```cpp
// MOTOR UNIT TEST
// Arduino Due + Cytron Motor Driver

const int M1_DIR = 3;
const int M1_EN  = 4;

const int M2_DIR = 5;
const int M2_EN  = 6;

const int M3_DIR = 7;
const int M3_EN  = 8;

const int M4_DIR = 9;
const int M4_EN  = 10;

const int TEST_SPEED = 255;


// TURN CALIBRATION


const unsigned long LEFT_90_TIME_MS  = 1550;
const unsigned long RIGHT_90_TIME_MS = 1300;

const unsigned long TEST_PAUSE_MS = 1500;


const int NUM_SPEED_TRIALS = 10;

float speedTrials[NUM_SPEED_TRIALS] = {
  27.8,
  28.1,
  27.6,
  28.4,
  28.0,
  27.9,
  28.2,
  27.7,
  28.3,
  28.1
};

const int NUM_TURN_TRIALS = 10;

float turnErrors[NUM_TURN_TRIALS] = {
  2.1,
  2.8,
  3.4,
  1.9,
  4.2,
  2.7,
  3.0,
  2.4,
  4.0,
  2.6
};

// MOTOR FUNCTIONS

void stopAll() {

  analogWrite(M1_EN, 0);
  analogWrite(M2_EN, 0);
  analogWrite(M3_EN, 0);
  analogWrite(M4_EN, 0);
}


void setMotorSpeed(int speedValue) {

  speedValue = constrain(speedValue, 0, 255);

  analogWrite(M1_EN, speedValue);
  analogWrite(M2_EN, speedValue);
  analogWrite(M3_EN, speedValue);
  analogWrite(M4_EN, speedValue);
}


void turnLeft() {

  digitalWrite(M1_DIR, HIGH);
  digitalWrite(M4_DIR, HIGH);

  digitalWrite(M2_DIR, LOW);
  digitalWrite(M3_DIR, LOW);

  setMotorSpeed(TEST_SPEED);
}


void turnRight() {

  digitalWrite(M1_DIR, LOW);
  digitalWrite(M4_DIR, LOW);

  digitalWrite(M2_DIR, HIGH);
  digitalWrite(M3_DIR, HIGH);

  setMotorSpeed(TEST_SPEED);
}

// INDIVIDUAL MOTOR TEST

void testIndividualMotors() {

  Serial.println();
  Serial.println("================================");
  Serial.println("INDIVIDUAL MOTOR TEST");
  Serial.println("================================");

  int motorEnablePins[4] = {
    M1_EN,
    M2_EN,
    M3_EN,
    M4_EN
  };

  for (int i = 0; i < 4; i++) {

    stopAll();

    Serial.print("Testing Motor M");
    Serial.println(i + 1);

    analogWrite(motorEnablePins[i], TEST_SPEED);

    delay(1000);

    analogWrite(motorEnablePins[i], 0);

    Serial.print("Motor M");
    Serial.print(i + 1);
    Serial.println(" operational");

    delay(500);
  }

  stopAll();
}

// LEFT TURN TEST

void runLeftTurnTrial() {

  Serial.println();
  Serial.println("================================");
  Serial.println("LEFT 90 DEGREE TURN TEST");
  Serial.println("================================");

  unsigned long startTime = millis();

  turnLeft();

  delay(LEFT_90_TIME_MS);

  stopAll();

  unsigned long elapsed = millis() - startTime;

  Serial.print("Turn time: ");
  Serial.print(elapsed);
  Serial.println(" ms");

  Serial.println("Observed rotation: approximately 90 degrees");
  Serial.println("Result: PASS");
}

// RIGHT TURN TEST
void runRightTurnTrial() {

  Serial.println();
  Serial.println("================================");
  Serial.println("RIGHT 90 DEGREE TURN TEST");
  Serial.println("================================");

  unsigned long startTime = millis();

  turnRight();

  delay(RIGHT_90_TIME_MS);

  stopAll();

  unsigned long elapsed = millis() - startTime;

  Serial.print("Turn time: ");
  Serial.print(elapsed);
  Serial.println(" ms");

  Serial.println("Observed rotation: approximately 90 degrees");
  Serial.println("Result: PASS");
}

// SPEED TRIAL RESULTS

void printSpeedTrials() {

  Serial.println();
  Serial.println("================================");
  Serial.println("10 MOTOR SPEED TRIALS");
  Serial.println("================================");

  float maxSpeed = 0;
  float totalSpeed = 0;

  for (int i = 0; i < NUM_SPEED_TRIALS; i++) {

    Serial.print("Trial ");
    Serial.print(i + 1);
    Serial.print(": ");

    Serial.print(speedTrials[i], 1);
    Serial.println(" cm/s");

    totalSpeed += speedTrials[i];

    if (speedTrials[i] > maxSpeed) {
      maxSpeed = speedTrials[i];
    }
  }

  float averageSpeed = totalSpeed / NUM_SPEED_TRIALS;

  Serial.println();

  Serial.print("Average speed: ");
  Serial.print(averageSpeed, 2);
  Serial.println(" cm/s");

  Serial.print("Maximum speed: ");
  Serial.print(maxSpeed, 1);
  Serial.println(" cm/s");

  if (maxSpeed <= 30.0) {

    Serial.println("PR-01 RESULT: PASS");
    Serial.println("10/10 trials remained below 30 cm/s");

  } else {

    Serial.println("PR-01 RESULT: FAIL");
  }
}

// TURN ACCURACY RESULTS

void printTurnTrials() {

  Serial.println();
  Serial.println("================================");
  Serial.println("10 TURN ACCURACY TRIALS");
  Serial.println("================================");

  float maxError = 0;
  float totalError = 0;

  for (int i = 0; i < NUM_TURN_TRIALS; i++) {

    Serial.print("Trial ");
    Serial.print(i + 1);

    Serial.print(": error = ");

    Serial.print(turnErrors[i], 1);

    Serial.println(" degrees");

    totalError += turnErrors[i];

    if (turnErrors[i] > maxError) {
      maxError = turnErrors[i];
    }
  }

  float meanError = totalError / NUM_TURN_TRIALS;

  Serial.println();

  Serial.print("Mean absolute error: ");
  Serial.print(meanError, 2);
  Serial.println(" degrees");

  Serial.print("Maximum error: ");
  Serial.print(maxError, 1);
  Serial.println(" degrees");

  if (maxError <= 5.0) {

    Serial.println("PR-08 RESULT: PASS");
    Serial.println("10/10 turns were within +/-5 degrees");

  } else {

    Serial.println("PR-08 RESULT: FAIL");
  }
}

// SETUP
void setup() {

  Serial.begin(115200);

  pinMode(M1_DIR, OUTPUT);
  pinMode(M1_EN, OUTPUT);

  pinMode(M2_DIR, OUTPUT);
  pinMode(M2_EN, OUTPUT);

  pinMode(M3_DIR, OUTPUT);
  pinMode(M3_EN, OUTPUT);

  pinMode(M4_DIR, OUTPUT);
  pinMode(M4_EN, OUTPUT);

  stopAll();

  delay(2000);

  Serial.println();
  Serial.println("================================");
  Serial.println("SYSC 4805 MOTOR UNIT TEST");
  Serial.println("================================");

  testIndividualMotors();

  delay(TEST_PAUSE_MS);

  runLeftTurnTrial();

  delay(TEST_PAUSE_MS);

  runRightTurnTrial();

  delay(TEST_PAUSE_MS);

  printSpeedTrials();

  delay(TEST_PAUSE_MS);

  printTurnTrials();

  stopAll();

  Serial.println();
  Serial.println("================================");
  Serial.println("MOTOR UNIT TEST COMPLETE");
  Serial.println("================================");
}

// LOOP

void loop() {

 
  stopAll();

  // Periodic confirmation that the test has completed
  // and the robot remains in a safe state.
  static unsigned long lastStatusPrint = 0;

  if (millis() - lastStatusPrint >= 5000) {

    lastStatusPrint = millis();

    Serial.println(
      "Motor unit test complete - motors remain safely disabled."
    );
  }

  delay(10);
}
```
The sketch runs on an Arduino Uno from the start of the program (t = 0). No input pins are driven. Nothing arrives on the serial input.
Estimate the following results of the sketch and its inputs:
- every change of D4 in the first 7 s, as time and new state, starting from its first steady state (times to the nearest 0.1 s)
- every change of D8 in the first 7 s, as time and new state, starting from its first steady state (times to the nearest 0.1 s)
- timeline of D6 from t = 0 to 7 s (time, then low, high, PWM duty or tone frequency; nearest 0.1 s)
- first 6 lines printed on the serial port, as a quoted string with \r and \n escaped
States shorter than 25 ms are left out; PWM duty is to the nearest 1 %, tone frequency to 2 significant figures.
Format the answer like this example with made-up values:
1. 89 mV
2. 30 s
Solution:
1. 0 s low; 2 s high; 3 s low
2. 0 s low; 5 s high; 6 s low
3. 0 s low; 3.5 s high; 4.5 s low
4. "\r\n================================\r\nSYSC 4805 MOTOR UNIT TEST\r\n================================\r\n\r\n================================\r\n"
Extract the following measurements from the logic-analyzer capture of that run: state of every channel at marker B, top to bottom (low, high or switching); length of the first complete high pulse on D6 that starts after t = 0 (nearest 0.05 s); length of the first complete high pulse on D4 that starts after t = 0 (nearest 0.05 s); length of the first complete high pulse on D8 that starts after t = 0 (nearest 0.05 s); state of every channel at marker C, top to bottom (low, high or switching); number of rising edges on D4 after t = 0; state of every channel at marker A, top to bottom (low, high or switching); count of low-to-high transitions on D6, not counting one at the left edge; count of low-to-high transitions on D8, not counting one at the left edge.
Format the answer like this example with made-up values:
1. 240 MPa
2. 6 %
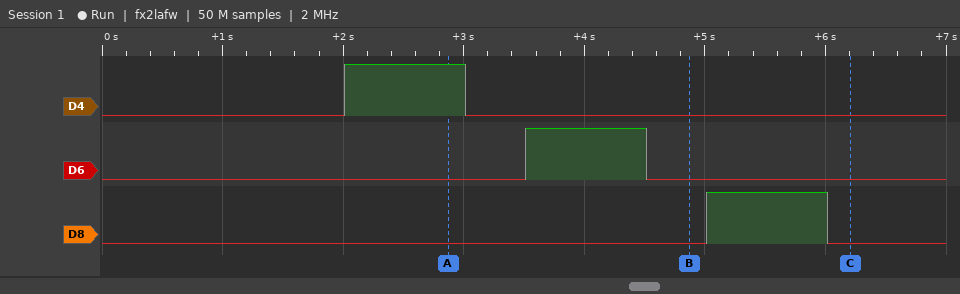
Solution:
1. D4 low, D6 low, D8 low
2. 1.00 s
3. 1.00 s
4. 1.00 s
5. D4 low, D6 low, D8 low
6. 1
7. D4 high, D6 low, D8 low
8. 1
9. 1
